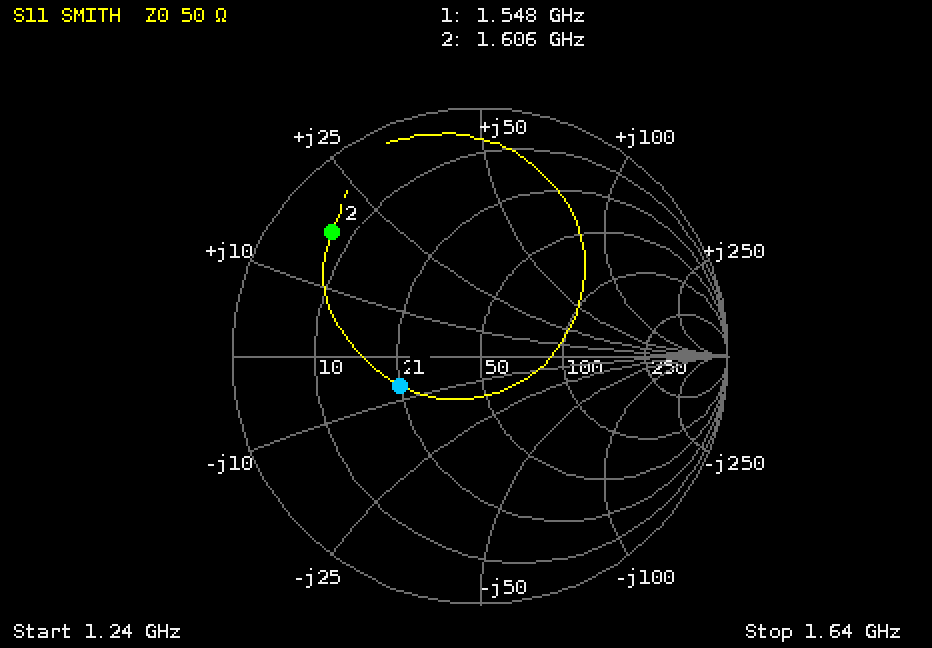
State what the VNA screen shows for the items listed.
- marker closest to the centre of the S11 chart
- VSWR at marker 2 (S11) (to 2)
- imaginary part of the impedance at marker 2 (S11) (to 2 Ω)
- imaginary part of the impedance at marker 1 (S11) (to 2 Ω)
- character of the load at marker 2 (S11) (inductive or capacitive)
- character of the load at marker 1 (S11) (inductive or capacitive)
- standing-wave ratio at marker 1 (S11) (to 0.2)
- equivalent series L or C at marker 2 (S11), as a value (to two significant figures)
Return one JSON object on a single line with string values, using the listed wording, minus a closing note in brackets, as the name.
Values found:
{"marker closest to the centre of the S11 chart": "marker 1", "VSWR at marker 2 (S11)": "8", "imaginary part of the impedance at marker 2 (S11)": "+18 Ω", "imaginary part of the impedance at marker 1 (S11)": "-6 Ω", "character of the load at marker 2 (S11)": "inductive", "character of the load at marker 1 (S11)": "capacitive", "standing-wave ratio at marker 1 (S11)": "2.0", "equivalent series L or C at marker 2 (S11), as a value": "1.8 nH"}
